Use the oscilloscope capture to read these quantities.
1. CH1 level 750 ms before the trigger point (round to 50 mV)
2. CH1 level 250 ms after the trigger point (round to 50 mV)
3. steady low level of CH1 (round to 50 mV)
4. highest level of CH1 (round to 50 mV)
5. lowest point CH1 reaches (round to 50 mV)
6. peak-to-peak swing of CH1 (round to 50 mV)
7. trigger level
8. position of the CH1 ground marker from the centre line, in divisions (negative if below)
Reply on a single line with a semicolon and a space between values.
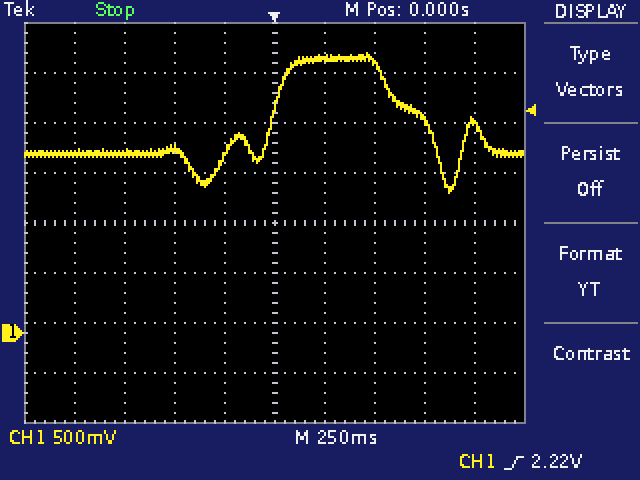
1.80 V; 2.75 V; 1.80 V; 2.80 V; 1.40 V; 1.40 V; 2.22 V; -2.2 div
